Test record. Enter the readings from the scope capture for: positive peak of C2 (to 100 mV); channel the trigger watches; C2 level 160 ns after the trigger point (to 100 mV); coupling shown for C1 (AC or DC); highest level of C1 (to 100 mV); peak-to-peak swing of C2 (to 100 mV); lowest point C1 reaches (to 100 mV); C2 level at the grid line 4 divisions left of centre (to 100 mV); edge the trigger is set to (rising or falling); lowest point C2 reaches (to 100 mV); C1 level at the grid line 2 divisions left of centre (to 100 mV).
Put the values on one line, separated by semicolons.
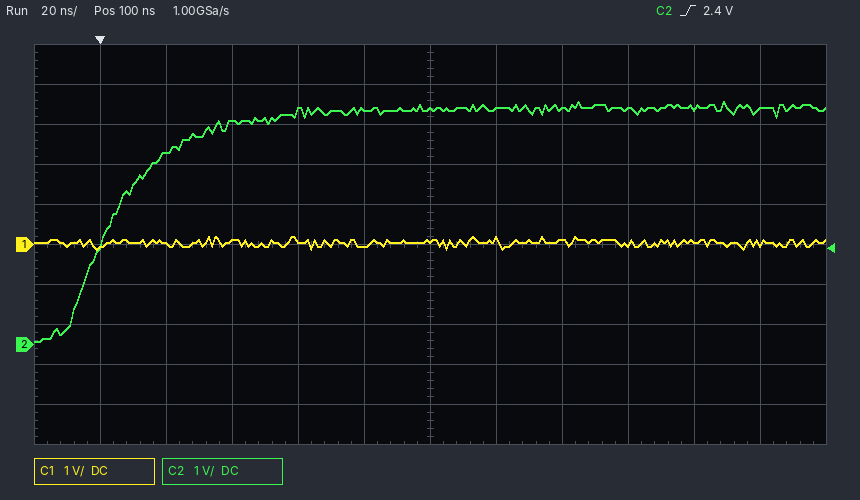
6.1 V; C2; 5.9 V; DC; 200 mV; 6.0 V; -100 mV; 4.8 V; rising; 100 mV; 100 mV
